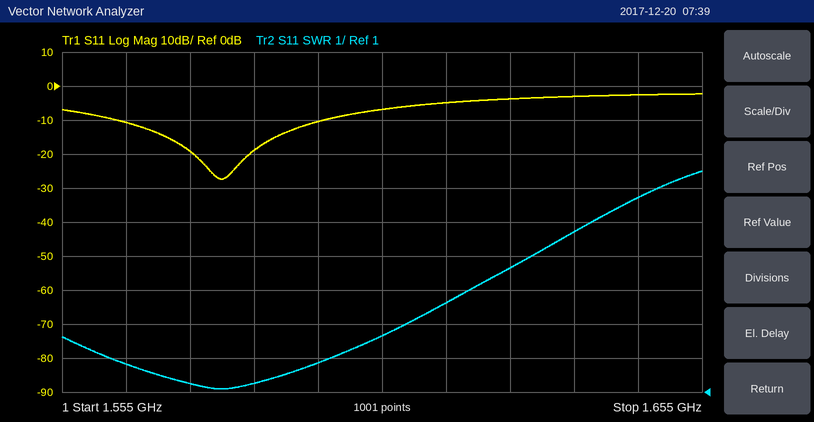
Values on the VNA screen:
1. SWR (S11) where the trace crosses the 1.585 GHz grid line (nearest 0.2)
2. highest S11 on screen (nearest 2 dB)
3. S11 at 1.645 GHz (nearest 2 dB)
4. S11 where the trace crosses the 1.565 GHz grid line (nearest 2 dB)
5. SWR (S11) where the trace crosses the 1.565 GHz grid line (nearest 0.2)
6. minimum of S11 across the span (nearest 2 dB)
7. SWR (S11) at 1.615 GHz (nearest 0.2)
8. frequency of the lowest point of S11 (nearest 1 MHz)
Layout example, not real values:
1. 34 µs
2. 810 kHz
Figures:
1. 1.2
2. -2 dB
3. -2 dB
4. -10 dB
5. 1.8
6. -28 dB
7. 3.6
8. 1.580 GHz
